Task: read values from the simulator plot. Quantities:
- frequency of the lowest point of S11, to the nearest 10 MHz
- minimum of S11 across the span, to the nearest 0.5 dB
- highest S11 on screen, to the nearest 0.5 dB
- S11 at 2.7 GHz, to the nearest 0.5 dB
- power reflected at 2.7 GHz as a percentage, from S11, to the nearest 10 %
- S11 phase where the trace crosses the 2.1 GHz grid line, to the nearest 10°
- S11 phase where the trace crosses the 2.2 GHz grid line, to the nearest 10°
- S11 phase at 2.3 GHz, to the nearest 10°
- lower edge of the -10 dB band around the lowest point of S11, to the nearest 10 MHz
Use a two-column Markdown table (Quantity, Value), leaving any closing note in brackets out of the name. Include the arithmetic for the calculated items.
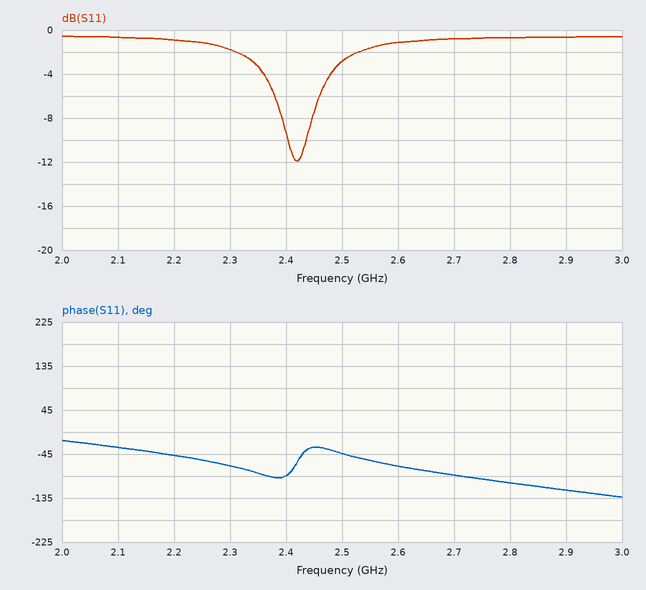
| Quantity | Value |
|---|---|
| frequency of the lowest point of S11, to the nearest 10 MHz | 2.42 GHz |
| minimum of S11 across the span, to the nearest 0.5 dB | -12.0 dB |
| highest S11 on screen, to the nearest 0.5 dB | -0.5 dB |
| S11 at 2.7 GHz, to the nearest 0.5 dB | -1.0 dB |
| power reflected at 2.7 GHz as a percentage, from S11, to the nearest 10 % | 10^(-1/10) ≈ 79.4 %, so 80 % to the nearest 10 % |
| S11 phase where the trace crosses the 2.1 GHz grid line, to the nearest 10° | -30° |
| S11 phase where the trace crosses the 2.2 GHz grid line, to the nearest 10° | -50° |
| S11 phase at 2.3 GHz, to the nearest 10° | -70° |
| lower edge of the -10 dB band around the lowest point of S11, to the nearest 10 MHz | 2.40 GHz |
